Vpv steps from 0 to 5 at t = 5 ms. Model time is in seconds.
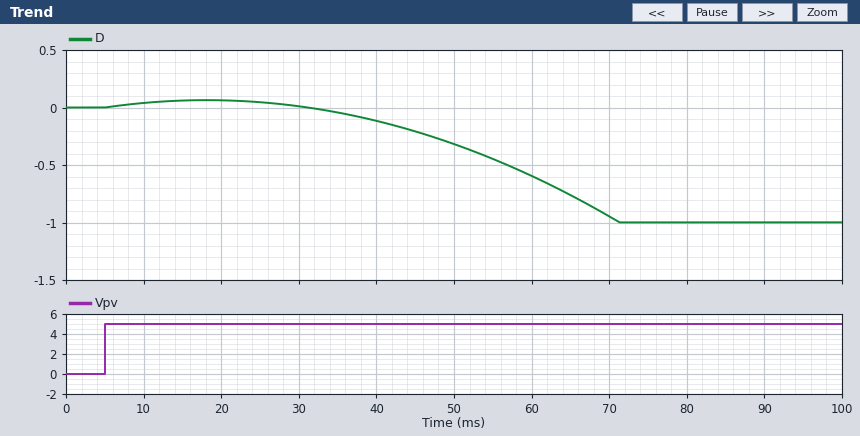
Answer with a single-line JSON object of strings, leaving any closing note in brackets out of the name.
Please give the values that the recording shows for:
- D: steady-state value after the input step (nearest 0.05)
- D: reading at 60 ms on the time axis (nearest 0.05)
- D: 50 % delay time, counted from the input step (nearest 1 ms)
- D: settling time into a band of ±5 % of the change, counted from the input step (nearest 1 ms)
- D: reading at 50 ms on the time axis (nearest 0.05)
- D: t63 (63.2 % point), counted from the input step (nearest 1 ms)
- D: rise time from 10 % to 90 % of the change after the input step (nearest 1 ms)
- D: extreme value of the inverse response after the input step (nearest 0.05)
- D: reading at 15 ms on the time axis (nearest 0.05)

{"D: steady-state value after the input step": "-1.00", "D: reading at 60 ms on the time axis": "-0.60", "D: 50 % delay time, counted from the input step": "52 ms", "D: settling time into a band of ±5 % of the change, counted from the input step": "65 ms", "D: reading at 50 ms on the time axis": "-0.30", "D: t63 (63.2 % point), counted from the input step": "56 ms", "D: rise time from 10 % to 90 % of the change after the input step": "30 ms", "D: extreme value of the inverse response after the input step": "0.05", "D: reading at 15 ms on the time axis": "0.05"}
